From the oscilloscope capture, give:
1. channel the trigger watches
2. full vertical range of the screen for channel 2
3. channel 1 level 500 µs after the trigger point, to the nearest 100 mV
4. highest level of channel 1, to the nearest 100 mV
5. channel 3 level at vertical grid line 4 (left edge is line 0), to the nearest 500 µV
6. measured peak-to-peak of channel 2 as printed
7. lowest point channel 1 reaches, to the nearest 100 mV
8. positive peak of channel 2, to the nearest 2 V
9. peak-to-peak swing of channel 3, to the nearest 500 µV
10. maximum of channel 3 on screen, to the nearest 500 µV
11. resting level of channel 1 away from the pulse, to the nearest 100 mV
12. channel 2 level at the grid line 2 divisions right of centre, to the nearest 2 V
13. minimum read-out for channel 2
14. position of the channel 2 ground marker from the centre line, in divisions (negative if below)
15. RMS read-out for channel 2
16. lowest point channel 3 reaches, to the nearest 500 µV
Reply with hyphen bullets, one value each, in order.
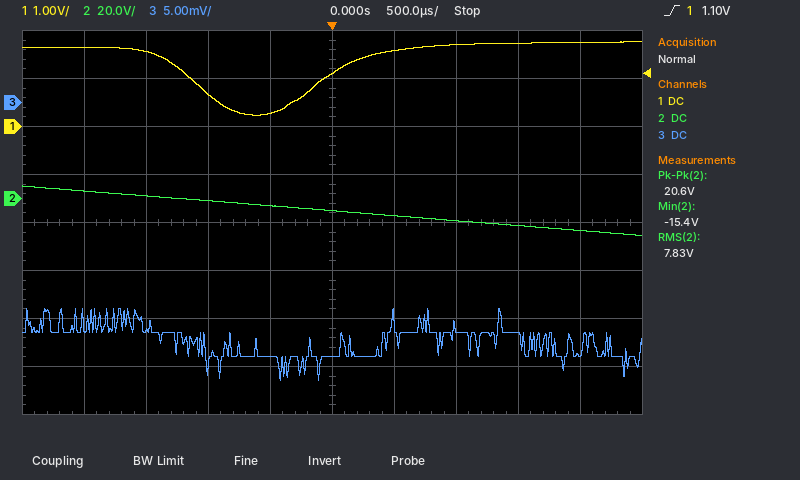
- channel 1
- 160 V
- 1.6 V
- 1.8 V
- -26.5 mV
- 20.6 V
- 200 mV
- 6 V
- 7.5 mV
- -21.5 mV
- 1.7 V
- -10 V
- -15.4 V
- +0.5 div
- 7.83 V
- -29.0 mV
